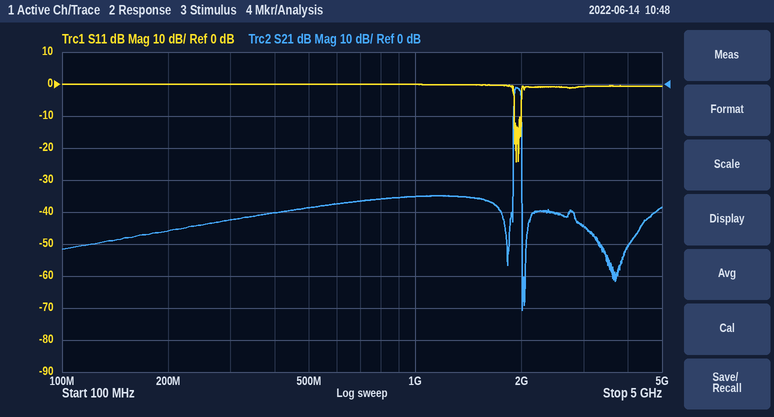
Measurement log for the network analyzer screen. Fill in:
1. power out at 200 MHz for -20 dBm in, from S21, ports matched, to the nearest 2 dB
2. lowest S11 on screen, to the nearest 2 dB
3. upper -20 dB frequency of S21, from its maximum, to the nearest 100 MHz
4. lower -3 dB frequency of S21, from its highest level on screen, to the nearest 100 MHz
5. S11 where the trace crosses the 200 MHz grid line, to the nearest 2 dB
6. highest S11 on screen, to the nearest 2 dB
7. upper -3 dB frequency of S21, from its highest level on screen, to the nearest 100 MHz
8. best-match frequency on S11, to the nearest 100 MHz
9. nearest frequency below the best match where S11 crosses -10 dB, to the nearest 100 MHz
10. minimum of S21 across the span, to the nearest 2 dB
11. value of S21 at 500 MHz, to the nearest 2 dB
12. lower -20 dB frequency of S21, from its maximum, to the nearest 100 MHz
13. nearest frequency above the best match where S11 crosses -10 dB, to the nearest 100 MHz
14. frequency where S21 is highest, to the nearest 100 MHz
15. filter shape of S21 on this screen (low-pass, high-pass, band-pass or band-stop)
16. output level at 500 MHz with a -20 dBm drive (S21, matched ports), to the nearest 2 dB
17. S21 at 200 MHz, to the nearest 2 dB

-66 dBm
-24 dB
2.0 GHz
1.9 GHz
0 dB
0 dB
2.0 GHz
1.9 GHz
1.9 GHz
-70 dB
-38 dB
1.9 GHz
2.0 GHz
1.9 GHz
band-pass
-58 dBm
-46 dB
